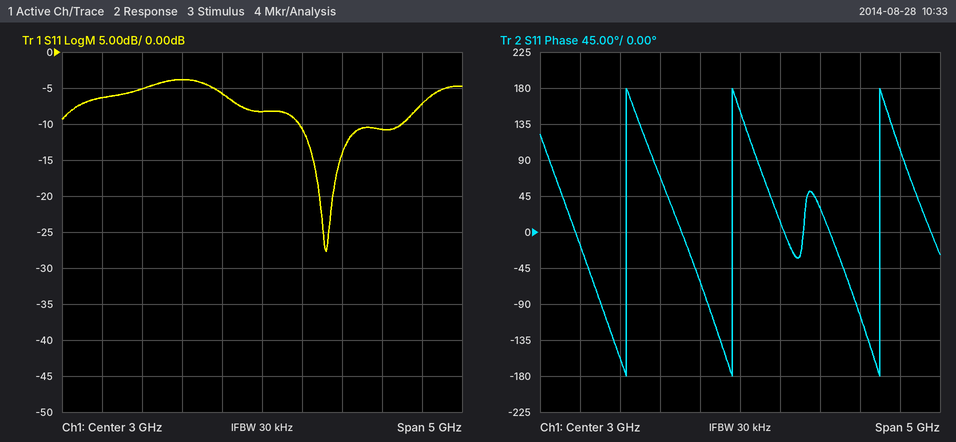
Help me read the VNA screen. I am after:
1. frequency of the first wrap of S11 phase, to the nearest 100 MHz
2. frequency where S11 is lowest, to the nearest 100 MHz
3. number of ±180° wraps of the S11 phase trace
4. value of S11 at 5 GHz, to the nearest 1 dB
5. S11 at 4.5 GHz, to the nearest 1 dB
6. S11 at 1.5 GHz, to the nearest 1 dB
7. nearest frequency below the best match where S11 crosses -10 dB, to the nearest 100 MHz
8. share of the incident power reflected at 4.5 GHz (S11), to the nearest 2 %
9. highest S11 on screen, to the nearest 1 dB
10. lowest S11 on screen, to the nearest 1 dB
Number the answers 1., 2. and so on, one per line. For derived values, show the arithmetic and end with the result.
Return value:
1. 1.6 GHz
2. 3.8 GHz
3. 3
4. -7 dB
5. -11 dB
6. -5 dB
7. 3.5 GHz
8. 10^(-11/10) ≈ 8 %
9. -4 dB
10. -28 dB
